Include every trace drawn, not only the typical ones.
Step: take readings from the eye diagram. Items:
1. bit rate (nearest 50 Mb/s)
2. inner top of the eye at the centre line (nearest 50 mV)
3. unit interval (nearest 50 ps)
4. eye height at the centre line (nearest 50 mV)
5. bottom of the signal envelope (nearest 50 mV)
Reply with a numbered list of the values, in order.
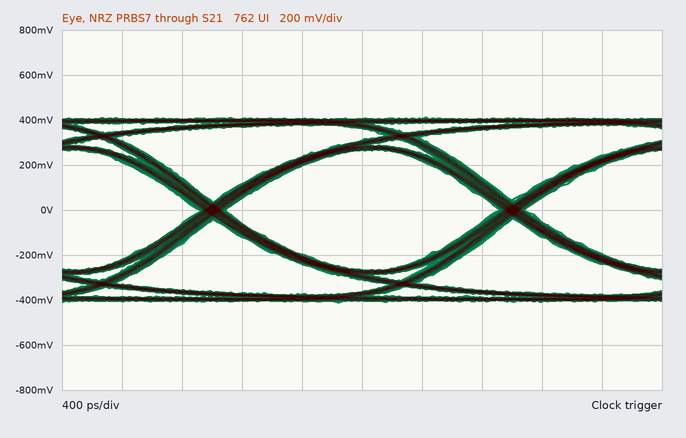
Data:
1. 500 Mb/s
2. 250 mV
3. 2.00 ns
4. 550 mV
5. -400 mV
